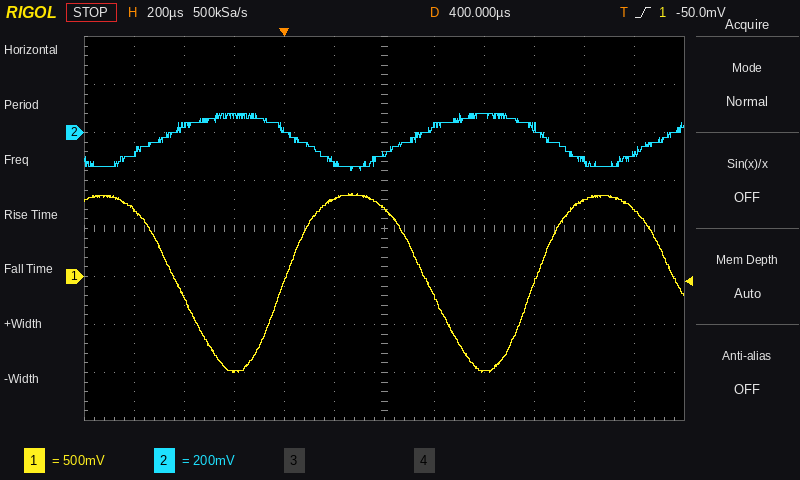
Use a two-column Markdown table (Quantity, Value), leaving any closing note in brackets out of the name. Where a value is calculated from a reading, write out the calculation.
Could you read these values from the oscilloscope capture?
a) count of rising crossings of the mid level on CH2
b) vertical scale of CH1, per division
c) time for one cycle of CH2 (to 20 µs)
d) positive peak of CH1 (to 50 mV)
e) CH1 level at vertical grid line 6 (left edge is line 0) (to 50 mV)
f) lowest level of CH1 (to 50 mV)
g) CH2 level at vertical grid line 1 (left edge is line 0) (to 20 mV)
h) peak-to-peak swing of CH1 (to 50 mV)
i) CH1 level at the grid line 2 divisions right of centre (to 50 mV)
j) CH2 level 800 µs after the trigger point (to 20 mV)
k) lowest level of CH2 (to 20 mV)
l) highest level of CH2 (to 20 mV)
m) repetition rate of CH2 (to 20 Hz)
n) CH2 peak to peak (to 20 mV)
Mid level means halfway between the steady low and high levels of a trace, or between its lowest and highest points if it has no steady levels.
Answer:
| Quantity | Value |
|---|---|
| count of rising crossings of the mid level on CH2 | 3 |
| vertical scale of CH1, per division | 500 mV |
| time for one cycle of CH2 | 1.00 ms |
| positive peak of CH1 | 850 mV |
| CH1 level at vertical grid line 6 (left edge is line 0) | 700 mV |
| lowest level of CH1 | -1.00 V |
| CH2 level at vertical grid line 1 (left edge is line 0) | -80 mV |
| peak-to-peak swing of CH1 | 850 mV − (-1.00 V) = 1.85 V |
| CH1 level at the grid line 2 divisions right of centre | -1.00 V |
| CH2 level 800 µs after the trigger point | 80 mV |
| lowest level of CH2 | -160 mV |
| highest level of CH2 | 80 mV |
| repetition rate of CH2 | 1 / 1.00 ms ≈ 1.00 kHz |
| CH2 peak to peak | 80 mV − (-160 mV) = 240 mV |
